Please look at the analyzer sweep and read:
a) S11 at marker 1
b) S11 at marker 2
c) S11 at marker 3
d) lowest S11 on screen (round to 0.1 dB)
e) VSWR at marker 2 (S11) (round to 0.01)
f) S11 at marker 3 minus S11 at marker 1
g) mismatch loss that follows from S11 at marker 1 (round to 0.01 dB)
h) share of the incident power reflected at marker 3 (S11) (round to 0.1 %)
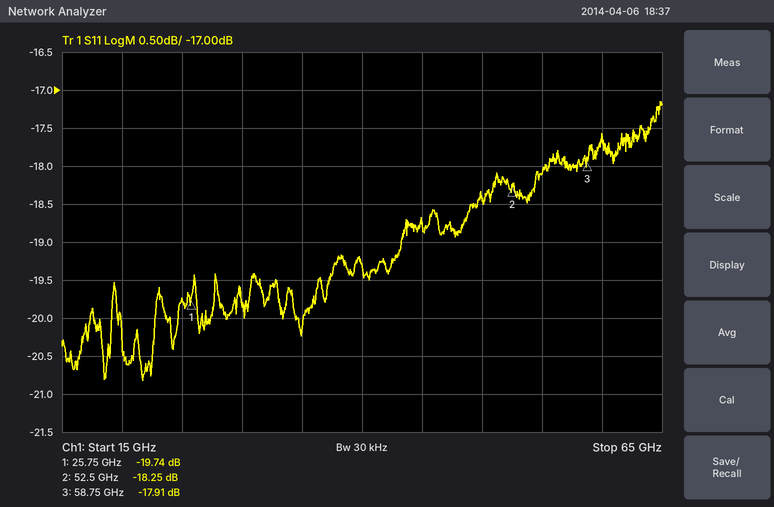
-19.74 dB
-18.25 dB
-17.91 dB
-20.8 dB
1.28
1.83 dB
0.05 dB
1.6 %
